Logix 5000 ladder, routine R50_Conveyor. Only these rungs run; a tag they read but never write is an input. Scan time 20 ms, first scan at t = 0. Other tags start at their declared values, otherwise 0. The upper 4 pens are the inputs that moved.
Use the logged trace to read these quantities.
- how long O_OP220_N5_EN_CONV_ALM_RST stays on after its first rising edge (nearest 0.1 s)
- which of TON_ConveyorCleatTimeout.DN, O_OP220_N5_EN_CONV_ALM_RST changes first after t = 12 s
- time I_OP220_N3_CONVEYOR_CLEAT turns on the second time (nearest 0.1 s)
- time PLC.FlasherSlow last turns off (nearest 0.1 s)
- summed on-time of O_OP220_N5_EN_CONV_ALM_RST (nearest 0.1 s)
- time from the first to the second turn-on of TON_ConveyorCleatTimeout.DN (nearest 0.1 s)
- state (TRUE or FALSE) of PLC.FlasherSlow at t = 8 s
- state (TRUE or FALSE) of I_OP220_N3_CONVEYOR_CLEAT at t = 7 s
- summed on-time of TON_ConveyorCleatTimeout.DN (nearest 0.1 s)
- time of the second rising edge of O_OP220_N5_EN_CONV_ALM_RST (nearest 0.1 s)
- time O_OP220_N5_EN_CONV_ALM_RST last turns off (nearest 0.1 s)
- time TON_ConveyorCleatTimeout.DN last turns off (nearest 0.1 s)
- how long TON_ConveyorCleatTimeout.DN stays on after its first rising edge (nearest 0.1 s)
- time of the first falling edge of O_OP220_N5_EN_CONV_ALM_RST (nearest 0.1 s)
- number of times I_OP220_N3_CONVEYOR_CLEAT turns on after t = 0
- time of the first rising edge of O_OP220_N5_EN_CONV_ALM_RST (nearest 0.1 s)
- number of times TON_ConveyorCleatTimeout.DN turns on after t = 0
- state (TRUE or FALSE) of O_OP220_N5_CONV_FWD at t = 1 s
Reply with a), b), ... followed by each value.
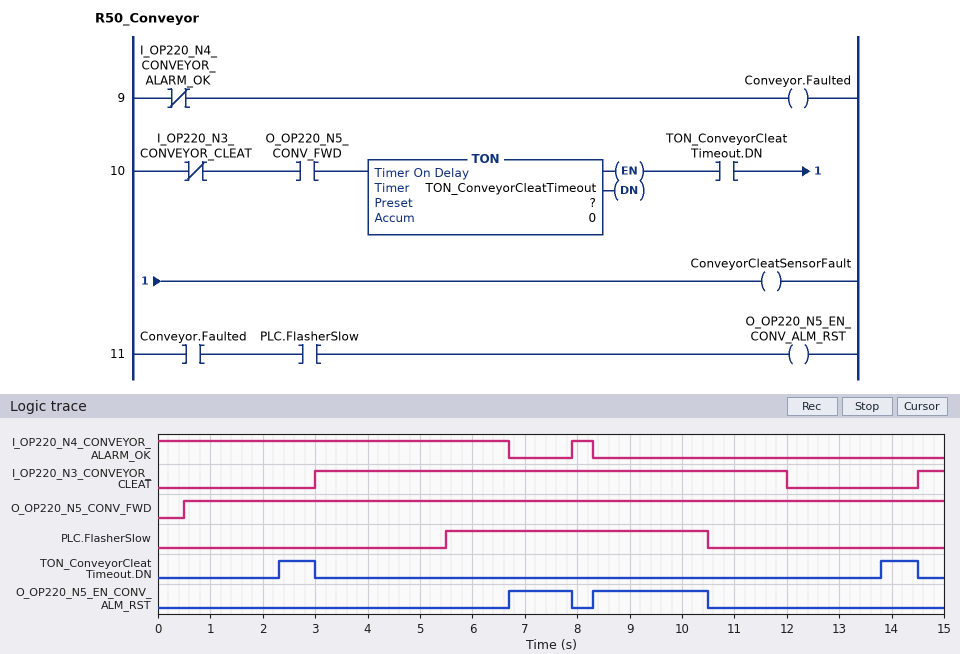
a) 1.2 s
b) TON_ConveyorCleatTimeout.DN
c) 14.5 s
d) 10.5 s
e) 3.4 s
f) 11.5 s
g) TRUE
h) TRUE
i) 1.4 s
j) 8.3 s
k) 10.5 s
l) 14.5 s
m) 0.7 s
n) 7.9 s
o) 2
p) 6.7 s
q) 2
r) TRUE
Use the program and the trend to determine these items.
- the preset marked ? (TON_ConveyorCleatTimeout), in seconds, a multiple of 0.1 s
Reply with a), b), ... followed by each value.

a) 1.8 s
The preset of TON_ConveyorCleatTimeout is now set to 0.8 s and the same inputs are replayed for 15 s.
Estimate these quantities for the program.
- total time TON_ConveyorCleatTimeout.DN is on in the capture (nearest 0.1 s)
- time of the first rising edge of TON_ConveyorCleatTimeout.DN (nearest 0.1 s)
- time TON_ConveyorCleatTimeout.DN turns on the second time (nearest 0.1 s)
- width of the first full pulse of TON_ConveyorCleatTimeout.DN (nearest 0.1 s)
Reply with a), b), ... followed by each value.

a) 3.4 s
b) 1.3 s
c) 12.8 s
d) 1.7 s
